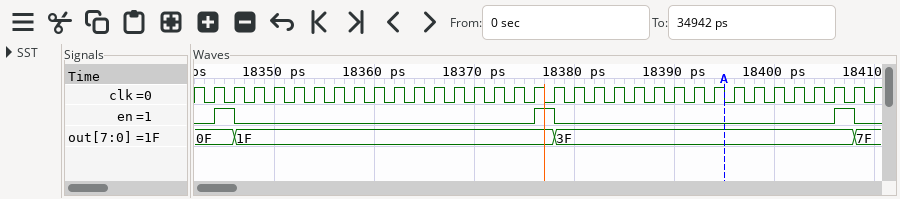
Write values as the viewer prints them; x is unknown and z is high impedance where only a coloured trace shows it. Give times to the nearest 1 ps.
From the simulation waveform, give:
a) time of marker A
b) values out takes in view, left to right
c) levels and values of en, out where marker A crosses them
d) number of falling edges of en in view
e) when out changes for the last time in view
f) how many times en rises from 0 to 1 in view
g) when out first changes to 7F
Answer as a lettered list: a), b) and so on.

a) 18395 ps
b) 0F, 1F, 3F, 7F
c) en=0, out=3F
d) 3
e) 18408 ps
f) 3
g) 18408 ps
